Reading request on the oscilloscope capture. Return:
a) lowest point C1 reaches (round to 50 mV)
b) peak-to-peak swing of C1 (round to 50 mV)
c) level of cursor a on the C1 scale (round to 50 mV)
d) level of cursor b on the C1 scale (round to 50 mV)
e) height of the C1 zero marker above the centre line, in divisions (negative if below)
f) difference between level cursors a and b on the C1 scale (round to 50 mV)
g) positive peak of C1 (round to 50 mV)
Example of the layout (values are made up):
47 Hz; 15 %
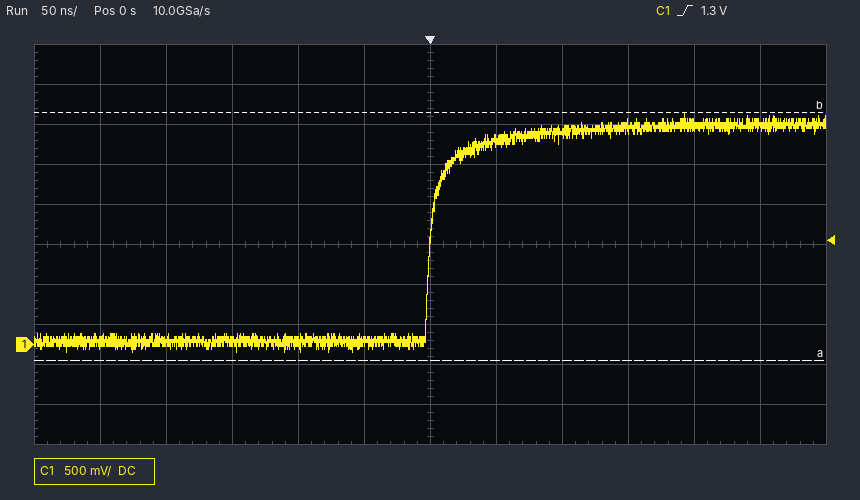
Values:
-100 mV; 3.00 V; -200 mV; 2.90 V; -2.5 div; 3.10 V; 2.90 V
